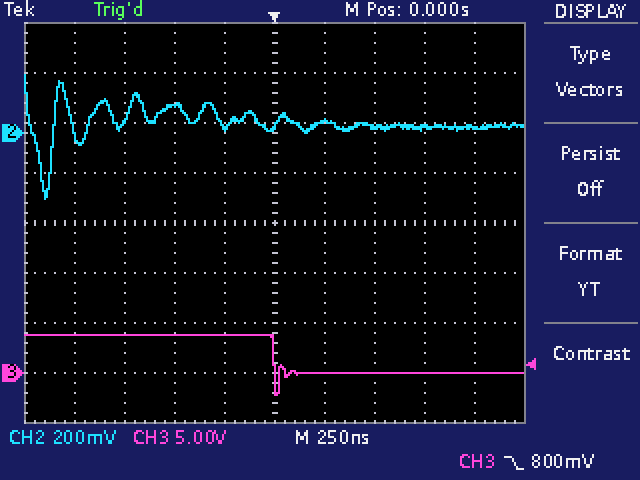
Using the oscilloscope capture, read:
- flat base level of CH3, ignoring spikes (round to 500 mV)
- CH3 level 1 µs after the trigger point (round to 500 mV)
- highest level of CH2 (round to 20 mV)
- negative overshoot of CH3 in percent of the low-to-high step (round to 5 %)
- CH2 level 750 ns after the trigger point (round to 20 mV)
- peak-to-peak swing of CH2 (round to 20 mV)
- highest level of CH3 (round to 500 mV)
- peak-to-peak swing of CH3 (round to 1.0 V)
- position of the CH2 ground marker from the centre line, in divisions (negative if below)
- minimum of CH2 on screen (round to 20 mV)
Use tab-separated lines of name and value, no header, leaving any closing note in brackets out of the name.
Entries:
flat base level of CH3, ignoring spikes	0.0 V
CH3 level 1 µs after the trigger point	0.0 V
highest level of CH2	240 mV
negative overshoot of CH3 in percent of the low-to-high step	60 %
CH2 level 750 ns after the trigger point	20 mV
peak-to-peak swing of CH2	500 mV
highest level of CH3	4.0 V
peak-to-peak swing of CH3	6.0 V
position of the CH2 ground marker from the centre line, in divisions	+1.8 div
minimum of CH2 on screen	-260 mV
